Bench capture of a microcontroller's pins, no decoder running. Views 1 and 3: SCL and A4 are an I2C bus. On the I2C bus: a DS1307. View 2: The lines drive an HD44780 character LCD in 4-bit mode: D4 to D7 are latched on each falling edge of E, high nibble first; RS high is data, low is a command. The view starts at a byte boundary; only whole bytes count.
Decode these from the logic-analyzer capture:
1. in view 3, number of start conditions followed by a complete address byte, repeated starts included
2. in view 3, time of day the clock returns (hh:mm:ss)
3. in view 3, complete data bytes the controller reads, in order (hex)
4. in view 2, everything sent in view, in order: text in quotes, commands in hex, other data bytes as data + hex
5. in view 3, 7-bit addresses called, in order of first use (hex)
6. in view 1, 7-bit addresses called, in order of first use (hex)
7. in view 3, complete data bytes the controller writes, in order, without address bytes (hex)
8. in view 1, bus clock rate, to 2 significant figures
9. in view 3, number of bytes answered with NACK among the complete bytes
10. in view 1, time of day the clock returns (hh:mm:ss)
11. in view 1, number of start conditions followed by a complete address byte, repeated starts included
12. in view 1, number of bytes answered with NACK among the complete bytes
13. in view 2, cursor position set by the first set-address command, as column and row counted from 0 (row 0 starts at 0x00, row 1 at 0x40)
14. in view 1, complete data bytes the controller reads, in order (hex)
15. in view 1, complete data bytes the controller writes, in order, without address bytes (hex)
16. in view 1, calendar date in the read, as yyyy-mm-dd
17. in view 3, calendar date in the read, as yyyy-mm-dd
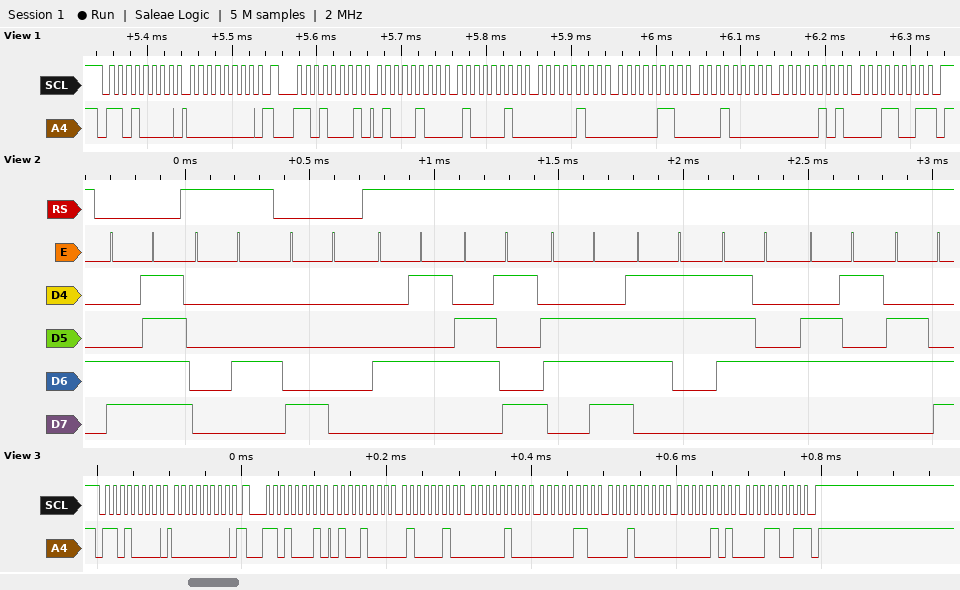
2
04:42:48
48 42 04 06 10 05 19
0xCF data 04 0x80 "Einstel"
0x68
0x68
00
100 kHz
1
04:42:44
2
1
column 15, row 1
44 42 04 06 10 05 19
00
2019-05-10
2019-05-10
